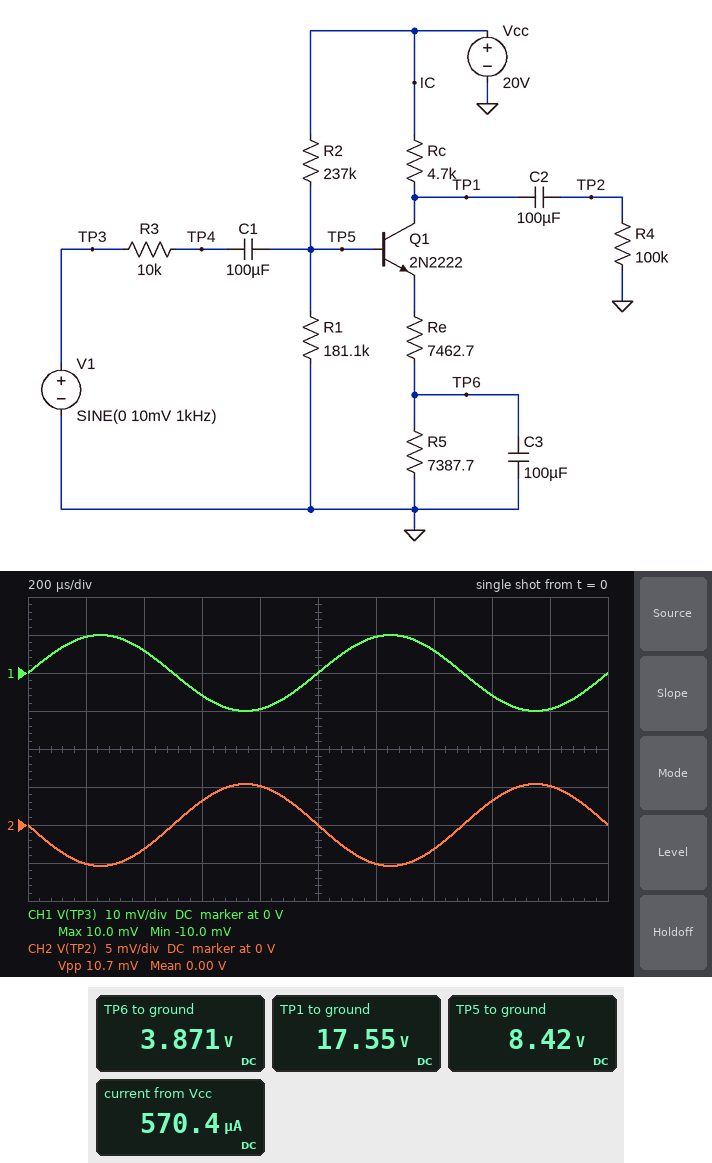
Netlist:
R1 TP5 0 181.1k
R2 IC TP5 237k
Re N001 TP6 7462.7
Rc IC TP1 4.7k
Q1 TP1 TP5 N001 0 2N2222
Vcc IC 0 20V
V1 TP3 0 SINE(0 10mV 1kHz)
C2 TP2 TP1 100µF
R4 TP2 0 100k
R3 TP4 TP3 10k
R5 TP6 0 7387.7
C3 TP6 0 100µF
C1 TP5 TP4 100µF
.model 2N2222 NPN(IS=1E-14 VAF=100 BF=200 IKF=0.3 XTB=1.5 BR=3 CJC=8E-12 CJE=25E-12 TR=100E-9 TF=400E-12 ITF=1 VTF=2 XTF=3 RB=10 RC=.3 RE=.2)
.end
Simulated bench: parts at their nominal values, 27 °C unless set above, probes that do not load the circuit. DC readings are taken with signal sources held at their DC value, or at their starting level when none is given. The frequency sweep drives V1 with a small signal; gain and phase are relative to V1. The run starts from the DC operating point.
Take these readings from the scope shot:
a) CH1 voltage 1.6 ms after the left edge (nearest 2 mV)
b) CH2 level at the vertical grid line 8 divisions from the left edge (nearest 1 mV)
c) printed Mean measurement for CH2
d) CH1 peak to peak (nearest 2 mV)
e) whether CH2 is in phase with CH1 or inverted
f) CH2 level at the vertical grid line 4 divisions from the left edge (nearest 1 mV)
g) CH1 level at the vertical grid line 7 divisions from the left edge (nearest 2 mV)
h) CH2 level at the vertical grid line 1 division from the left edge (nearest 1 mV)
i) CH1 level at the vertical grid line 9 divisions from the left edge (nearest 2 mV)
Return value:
-6 mV
3 mV
0.00 V
20 mV
inverted
5 mV
6 mV
-5 mV
-10 mV
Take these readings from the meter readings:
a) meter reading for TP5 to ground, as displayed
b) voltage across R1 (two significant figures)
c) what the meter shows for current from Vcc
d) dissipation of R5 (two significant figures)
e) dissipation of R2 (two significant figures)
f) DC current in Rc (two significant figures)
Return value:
8.42 V
8.4 V
570.4 µA
2.0 mW
570 µW
520 µA
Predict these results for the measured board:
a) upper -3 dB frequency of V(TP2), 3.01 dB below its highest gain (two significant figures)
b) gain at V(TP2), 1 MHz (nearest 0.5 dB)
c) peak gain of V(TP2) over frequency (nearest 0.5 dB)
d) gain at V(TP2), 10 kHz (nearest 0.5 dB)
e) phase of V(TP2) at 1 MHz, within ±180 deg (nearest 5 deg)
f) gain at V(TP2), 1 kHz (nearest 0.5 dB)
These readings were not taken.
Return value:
2.9 MHz
-6.0 dB
-5.5 dB
-5.5 dB
145 deg
-5.5 dB
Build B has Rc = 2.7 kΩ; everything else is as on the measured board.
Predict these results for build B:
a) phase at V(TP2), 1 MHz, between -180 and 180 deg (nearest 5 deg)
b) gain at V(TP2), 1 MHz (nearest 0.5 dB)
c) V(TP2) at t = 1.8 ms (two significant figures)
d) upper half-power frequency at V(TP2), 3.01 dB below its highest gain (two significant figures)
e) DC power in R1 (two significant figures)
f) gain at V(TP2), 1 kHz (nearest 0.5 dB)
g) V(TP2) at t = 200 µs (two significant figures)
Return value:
150 deg
-10.5 dB
3.0 mV
4.5 MHz
390 µW
-10.0 dB
-3.0 mV
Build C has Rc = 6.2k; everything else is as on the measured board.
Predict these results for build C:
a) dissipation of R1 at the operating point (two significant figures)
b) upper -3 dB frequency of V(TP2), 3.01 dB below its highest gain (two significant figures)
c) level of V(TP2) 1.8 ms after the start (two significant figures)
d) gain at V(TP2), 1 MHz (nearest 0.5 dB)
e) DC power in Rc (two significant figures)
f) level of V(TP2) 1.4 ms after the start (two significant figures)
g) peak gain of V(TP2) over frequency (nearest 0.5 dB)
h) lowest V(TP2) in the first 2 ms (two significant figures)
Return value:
390 µW
2.3 MHz
6.7 mV
-4.0 dB
1.7 mW
-4.1 mV
-3.0 dB
-7.0 mV
